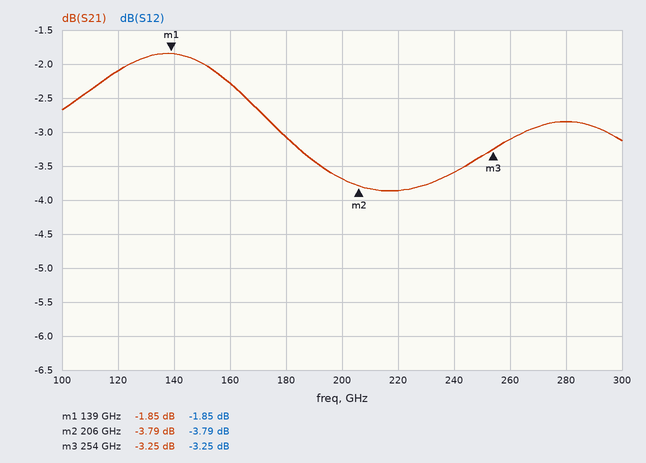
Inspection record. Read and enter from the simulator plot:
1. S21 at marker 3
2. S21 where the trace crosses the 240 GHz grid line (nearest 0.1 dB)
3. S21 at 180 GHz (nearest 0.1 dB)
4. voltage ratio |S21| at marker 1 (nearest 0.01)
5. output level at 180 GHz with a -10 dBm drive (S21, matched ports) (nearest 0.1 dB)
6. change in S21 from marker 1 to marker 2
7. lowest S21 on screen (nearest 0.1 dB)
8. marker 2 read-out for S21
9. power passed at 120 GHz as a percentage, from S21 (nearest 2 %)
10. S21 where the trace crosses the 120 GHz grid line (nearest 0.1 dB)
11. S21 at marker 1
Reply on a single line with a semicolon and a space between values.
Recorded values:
-3.25 dB; -3.6 dB; -3.1 dB; 0.81; -13.1 dBm; -1.94 dB; -3.9 dB; -3.79 dB; 62 %; -2.1 dB; -1.85 dB
